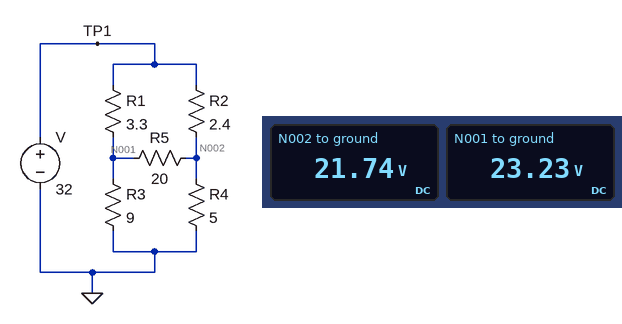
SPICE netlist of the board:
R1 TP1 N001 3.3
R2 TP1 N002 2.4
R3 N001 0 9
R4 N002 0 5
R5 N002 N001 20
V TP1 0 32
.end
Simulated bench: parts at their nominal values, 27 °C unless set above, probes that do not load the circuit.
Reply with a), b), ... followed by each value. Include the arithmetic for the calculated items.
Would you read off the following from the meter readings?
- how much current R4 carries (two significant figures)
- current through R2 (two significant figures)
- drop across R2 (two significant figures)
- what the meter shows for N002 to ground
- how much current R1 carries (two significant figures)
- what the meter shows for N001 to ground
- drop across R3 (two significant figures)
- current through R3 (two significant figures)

a) (21.74 V) / 5 Ω = 4.3 A
b) (32 V - 21.74 V) / 2.4 Ω = 4.3 A
c) 32 V - 21.74 V = 10 V
d) 21.74 V
e) (32 V - 23.23 V) / 3.3 Ω = 2.7 A
f) 23.23 V
g) 23.23 V = 23 V
h) (23.23 V) / 9 Ω = 2.6 A
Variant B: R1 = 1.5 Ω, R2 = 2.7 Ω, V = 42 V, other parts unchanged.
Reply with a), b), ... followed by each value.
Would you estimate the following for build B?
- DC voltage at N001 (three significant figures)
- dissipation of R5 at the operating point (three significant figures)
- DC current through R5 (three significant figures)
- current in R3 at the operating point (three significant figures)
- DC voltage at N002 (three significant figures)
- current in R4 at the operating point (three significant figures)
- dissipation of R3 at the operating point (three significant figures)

a) 35.5 V
b) 2.87 W
c) 379 mA
d) 3.95 A
e) 27.9 V
f) 5.59 A
g) 140 W
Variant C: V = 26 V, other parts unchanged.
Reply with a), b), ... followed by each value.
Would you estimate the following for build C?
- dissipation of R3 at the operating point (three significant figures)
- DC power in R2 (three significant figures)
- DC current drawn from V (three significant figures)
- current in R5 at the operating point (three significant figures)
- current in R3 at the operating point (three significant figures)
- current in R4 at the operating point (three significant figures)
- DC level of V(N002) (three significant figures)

a) 39.6 W
b) 28.9 W
c) 5.63 A
d) 60.6 mA
e) 2.10 A
f) 3.53 A
g) 17.7 V
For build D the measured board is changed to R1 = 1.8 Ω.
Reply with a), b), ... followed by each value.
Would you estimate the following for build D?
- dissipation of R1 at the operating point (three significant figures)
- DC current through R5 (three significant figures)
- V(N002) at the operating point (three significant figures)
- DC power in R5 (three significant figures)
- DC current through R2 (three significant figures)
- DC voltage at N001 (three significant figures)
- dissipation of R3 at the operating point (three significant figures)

a) 17.8 W
b) 218 mA
c) 22.0 V
d) 952 mW
e) 4.18 A
f) 26.3 V
g) 77.1 W
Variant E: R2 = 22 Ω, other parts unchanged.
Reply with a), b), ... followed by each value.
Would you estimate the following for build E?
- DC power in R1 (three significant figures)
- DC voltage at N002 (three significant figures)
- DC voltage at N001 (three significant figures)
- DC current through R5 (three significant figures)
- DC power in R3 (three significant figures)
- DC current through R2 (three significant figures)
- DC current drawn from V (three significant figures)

a) 31.4 W
b) 8.62 V
c) 21.8 V
d) 660 mA
e) 52.9 W
f) 1.06 A
g) 4.15 A
